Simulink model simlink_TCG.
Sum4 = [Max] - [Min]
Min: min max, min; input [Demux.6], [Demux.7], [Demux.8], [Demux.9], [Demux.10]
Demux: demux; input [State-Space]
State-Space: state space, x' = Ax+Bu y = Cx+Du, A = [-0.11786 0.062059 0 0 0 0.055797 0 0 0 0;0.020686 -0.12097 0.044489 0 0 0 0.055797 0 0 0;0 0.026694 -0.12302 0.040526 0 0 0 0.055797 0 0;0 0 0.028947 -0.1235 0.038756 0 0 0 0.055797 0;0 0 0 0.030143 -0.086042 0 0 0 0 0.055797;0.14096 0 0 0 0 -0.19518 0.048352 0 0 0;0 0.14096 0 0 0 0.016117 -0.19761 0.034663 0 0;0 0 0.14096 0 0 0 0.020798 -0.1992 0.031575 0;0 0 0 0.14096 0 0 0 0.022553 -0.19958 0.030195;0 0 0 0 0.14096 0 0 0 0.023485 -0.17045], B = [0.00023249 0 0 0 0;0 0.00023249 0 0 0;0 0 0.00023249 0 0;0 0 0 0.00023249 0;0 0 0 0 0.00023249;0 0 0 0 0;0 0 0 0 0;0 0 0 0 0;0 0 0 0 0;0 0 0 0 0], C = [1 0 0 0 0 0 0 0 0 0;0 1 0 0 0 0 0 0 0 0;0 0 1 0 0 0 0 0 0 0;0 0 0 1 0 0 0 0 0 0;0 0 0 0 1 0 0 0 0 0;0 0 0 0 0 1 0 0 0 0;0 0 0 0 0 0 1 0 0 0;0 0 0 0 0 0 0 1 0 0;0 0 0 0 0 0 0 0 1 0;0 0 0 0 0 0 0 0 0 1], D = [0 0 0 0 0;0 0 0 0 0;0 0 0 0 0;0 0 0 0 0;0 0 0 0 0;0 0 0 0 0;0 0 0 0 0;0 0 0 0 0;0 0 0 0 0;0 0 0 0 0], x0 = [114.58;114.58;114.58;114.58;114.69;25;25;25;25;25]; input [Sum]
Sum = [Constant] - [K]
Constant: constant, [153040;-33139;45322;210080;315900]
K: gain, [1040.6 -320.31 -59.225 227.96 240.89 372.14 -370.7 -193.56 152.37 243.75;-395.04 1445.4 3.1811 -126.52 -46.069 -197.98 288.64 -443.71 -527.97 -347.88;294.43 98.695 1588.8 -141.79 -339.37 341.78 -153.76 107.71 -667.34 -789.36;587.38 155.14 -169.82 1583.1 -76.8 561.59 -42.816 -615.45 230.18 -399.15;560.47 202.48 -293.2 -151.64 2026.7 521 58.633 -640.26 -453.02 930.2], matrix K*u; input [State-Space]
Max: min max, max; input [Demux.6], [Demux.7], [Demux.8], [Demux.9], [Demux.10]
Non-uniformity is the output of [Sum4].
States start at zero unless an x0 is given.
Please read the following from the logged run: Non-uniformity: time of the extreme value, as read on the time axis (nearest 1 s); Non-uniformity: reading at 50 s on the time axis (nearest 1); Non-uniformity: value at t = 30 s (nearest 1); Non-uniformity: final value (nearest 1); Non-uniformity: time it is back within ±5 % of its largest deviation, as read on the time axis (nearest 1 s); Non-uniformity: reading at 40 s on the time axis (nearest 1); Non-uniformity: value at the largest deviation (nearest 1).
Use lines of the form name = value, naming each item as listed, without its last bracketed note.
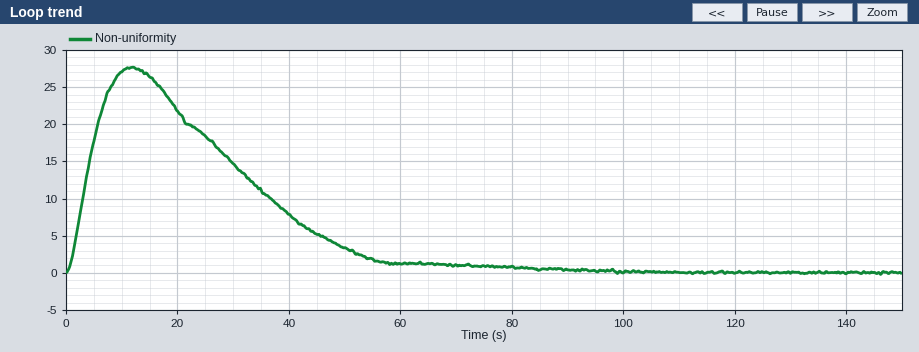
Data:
Non-uniformity: time of the extreme value, as read on the time axis = 12 s
Non-uniformity: reading at 50 s on the time axis = 3
Non-uniformity: value at t = 30 s = 15
Non-uniformity: final value = 0
Non-uniformity: time it is back within ±5 % of its largest deviation, as read on the time axis = 57 s
Non-uniformity: reading at 40 s on the time axis = 8
Non-uniformity: value at the largest deviation = 28
